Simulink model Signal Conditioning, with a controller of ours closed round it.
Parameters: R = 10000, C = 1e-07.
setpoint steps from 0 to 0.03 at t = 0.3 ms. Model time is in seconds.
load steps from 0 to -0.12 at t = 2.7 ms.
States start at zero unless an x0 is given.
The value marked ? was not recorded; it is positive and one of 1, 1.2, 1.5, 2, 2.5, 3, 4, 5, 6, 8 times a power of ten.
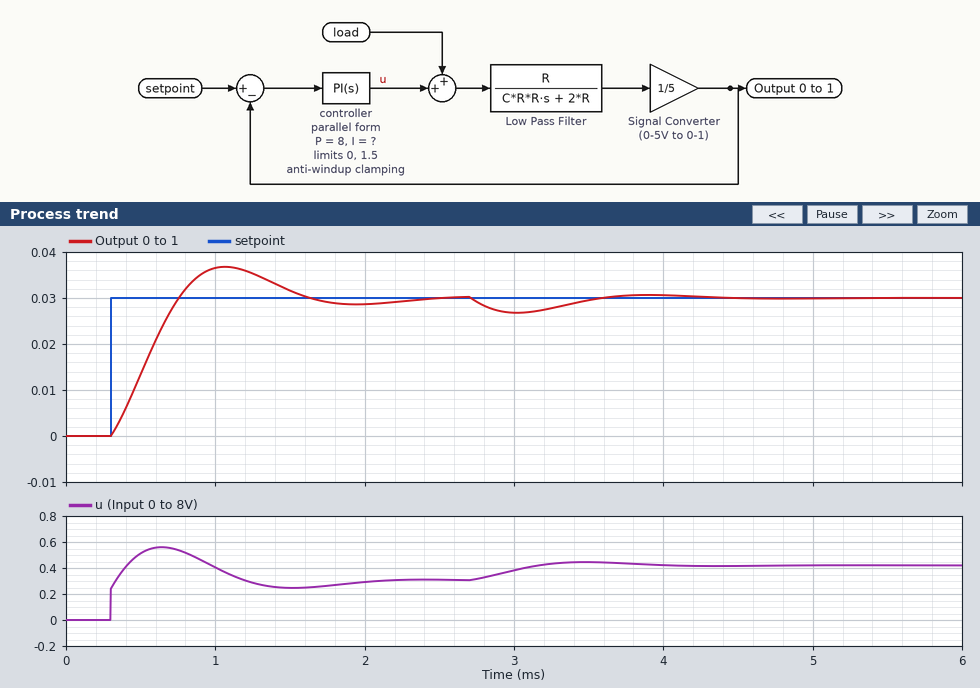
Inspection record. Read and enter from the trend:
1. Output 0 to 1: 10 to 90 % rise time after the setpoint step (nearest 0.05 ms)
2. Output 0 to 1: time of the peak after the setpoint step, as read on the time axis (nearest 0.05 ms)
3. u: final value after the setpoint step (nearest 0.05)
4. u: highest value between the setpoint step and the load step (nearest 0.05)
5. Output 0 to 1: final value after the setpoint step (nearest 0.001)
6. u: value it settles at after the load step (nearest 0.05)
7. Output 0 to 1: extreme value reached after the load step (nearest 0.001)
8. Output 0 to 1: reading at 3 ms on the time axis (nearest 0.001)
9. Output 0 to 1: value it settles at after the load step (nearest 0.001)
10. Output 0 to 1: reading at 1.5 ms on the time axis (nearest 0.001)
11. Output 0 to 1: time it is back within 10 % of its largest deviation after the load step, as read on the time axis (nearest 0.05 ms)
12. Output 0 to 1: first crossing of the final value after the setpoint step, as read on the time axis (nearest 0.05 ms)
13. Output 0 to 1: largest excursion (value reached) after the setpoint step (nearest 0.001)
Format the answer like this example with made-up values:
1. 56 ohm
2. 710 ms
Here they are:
1. 0.35 ms
2. 1.05 ms
3. 0.30
4. 0.55
5. 0.030
6. 0.40
7. 0.027
8. 0.027
9. 0.030
10. 0.032
11. 4.20 ms
12. 0.75 ms
13. 0.037
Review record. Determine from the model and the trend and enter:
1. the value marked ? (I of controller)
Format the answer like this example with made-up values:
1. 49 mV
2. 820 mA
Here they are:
1. 80000
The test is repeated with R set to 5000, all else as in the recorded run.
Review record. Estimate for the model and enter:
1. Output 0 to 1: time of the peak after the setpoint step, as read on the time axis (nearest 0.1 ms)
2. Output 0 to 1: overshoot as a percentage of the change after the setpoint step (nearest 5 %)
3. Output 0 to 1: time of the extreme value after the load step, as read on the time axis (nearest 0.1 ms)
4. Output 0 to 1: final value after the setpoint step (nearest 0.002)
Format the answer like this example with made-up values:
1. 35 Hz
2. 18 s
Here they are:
1. 0.9 ms
2. 10 %
3. 2.9 ms
4. 0.030
